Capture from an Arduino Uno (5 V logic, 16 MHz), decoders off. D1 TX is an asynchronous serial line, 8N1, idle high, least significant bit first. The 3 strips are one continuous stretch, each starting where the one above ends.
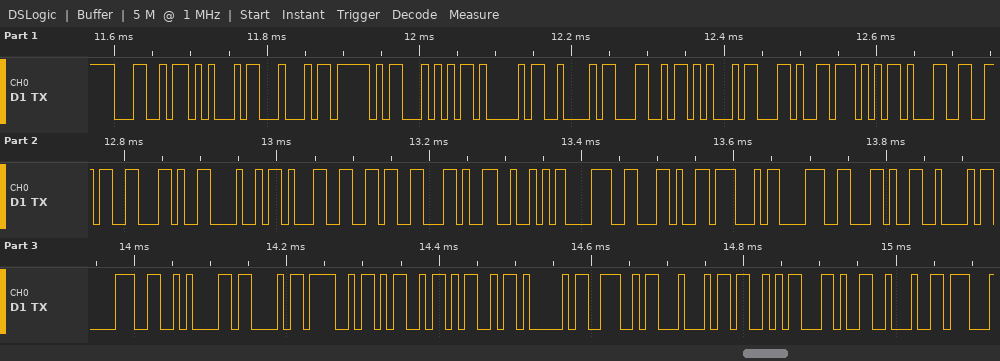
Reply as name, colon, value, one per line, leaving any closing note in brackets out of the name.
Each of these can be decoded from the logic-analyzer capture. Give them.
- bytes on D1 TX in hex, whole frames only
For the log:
bytes on D1 TX in hex, whole frames only: 4C 45 44 5F 54 41 42 4C 45 2C 57 31 36 2C 48 31 36 2C 52 38 2C 47 38 2C 42 38 0A 43 4F 4D 4D 41 4E 44 53 2C 22
